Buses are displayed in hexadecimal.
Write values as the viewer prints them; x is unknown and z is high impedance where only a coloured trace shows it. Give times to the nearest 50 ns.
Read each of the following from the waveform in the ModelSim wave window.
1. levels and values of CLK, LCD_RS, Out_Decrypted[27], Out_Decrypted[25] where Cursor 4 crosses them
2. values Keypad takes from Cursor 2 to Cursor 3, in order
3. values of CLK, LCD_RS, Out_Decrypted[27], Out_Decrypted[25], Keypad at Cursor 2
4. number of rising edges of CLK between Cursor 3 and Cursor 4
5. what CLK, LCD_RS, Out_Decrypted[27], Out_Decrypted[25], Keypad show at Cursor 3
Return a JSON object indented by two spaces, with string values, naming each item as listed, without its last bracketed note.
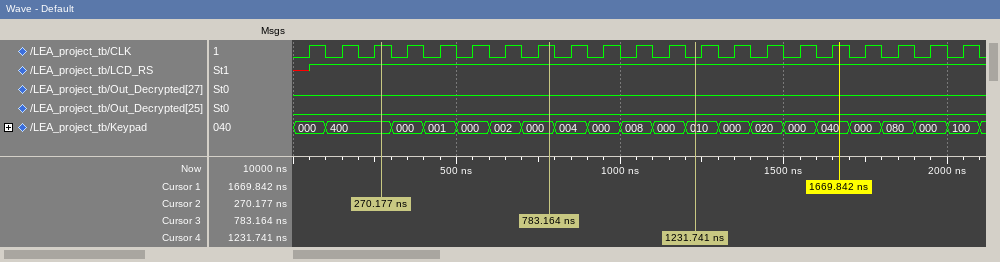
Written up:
{
  "levels and values of CLK, LCD_RS, Out_Decrypted[27], Out_Decrypted[25] where Cursor 4 crosses them": "CLK=0, LCD_RS=1, Out_Decrypted[27]=0, Out_Decrypted[25]=0",
  "values Keypad takes from Cursor 2 to Cursor 3, in order": "400, 000, 001, 000, 002, 000",
  "values of CLK, LCD_RS, Out_Decrypted[27], Out_Decrypted[25], Keypad at Cursor 2": "CLK=1, LCD_RS=1, Out_Decrypted[27]=0, Out_Decrypted[25]=0, Keypad=400",
  "number of rising edges of CLK between Cursor 3 and Cursor 4": "4",
  "what CLK, LCD_RS, Out_Decrypted[27], Out_Decrypted[25], Keypad show at Cursor 3": "CLK=1, LCD_RS=1, Out_Decrypted[27]=0, Out_Decrypted[25]=0, Keypad=000"
}
